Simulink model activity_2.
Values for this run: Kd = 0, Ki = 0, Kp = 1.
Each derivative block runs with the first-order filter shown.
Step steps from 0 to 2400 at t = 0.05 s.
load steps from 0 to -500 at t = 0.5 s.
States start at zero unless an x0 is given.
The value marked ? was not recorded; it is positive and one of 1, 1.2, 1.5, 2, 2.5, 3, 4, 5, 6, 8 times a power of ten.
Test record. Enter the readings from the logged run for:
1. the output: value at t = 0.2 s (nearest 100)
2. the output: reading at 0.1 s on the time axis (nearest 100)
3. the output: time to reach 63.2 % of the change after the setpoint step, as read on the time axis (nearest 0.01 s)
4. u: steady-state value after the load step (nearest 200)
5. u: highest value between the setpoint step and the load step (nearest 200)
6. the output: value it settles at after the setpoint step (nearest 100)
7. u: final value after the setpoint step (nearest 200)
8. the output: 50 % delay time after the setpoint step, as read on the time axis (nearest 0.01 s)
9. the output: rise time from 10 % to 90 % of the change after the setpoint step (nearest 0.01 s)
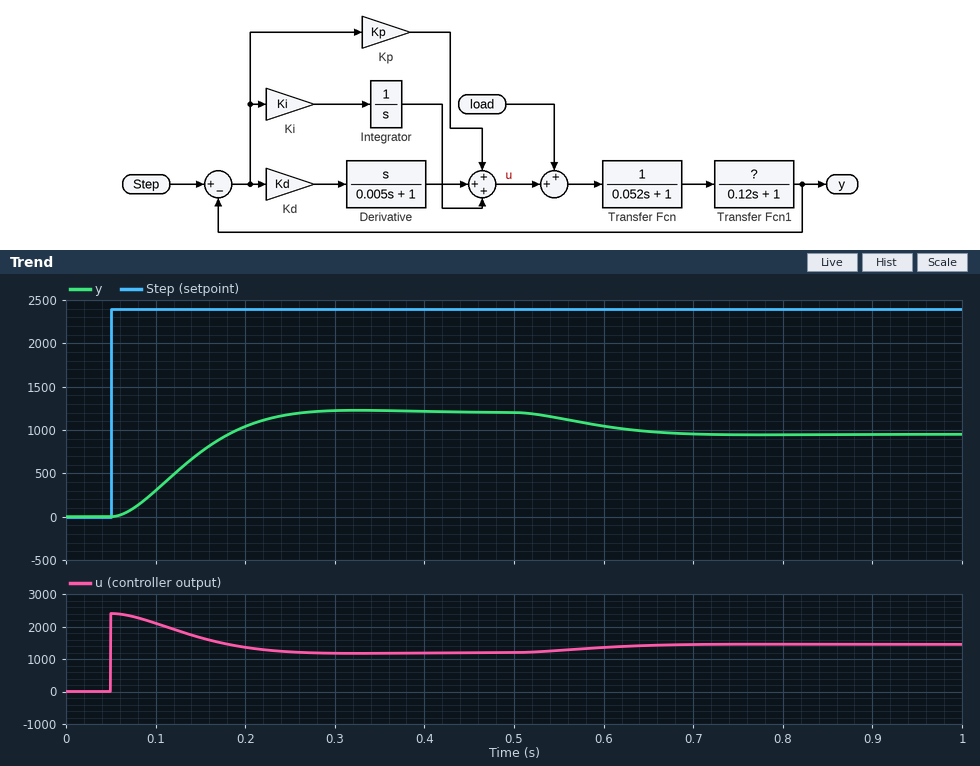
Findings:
1000
300
0.15 s
1400
2400
1200
1200
0.13 s
0.13 s
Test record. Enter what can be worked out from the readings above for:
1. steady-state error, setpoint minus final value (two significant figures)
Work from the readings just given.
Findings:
1200
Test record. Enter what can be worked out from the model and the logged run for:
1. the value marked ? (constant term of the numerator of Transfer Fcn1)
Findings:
1
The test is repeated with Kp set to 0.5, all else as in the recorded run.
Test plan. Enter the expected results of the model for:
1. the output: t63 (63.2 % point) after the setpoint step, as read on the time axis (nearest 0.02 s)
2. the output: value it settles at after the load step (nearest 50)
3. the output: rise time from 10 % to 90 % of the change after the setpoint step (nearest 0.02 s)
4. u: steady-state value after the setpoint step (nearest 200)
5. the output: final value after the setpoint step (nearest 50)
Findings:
0.18 s
450
0.18 s
800
800
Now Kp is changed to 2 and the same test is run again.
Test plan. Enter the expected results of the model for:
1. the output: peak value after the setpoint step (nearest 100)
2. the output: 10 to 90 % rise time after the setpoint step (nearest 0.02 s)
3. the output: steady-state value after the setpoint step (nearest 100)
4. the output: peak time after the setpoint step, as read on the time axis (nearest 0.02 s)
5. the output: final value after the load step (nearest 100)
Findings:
1700
0.08 s
1600
0.24 s
1400
